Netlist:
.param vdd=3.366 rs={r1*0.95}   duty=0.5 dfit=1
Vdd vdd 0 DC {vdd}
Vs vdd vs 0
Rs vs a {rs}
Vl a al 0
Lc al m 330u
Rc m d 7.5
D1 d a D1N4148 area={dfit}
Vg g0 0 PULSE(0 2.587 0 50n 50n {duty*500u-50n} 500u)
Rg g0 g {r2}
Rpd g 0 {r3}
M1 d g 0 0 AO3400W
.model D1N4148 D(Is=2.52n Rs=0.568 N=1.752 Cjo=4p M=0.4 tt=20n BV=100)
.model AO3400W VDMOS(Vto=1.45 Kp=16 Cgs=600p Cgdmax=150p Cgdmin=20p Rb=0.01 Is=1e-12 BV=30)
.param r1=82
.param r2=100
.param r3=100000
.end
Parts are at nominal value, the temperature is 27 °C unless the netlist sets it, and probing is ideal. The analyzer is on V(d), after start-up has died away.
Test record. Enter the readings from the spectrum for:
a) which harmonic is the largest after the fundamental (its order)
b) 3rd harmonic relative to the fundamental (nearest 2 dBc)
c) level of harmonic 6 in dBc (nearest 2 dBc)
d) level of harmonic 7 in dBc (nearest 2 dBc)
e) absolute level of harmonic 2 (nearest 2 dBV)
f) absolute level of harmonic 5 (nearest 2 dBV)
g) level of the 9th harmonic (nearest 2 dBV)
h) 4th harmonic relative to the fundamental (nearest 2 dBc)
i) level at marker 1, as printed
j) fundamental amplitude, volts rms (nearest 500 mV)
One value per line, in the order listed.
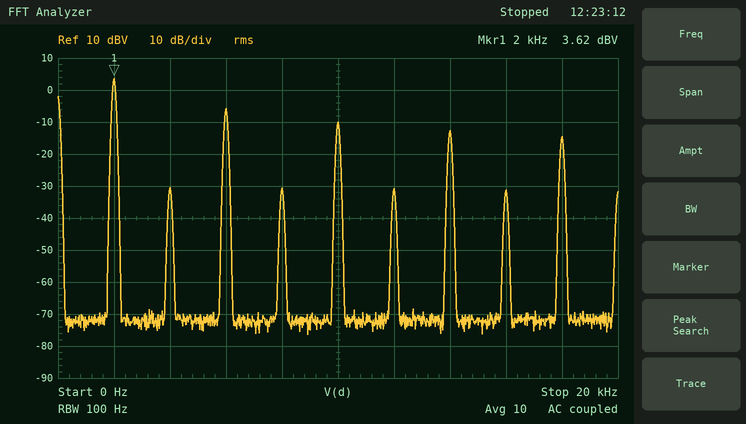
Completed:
3
-10 dBc
-34 dBc
-16 dBc
-30 dBV
-10 dBV
-14 dBV
-34 dBc
3.62 dBV
1.5 V
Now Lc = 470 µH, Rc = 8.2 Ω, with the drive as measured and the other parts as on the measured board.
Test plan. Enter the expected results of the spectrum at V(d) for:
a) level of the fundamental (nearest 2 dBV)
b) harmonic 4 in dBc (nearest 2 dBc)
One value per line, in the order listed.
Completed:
4 dBV
-32 dBc
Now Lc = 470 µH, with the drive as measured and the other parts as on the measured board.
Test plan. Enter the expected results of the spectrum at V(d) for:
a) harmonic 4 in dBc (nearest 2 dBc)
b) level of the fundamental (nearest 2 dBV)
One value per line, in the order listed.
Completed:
-32 dBc
4 dBV
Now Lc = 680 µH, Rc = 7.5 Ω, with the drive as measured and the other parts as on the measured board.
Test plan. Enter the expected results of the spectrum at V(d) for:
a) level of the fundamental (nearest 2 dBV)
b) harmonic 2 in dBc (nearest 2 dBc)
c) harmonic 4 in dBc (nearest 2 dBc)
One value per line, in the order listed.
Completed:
4 dBV
-28 dBc
-28 dBc
